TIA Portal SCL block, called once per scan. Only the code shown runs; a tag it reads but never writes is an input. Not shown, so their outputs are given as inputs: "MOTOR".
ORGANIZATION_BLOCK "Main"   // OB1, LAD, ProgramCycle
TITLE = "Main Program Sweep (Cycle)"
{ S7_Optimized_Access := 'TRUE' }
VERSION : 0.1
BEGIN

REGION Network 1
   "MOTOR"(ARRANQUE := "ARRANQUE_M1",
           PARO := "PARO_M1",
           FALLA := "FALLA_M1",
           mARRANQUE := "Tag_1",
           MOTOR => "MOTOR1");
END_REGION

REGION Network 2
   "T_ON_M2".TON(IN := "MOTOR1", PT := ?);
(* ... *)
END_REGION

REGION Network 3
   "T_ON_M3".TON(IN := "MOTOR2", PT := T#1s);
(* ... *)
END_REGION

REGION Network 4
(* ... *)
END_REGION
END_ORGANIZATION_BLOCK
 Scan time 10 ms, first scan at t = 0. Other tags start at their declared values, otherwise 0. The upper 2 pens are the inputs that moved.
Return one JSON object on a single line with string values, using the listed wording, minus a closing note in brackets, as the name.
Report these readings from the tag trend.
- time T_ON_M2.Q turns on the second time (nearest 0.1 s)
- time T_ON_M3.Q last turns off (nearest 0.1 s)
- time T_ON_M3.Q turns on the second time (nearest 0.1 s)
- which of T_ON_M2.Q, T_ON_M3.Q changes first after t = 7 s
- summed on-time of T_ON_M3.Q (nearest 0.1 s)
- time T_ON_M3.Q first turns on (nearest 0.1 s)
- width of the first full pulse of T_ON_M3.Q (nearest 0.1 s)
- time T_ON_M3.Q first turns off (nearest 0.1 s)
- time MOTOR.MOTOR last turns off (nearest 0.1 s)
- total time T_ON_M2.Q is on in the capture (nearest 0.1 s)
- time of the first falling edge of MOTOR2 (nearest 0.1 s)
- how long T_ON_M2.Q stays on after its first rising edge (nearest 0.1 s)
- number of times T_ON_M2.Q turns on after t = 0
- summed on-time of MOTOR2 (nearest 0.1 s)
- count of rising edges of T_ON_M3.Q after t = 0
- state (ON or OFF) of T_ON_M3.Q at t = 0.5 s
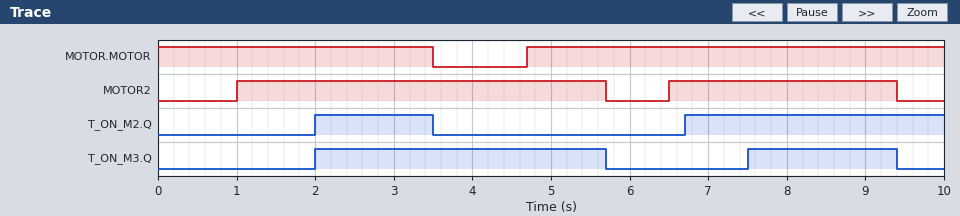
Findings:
{"time T_ON_M2.Q turns on the second time": "6.7 s", "time T_ON_M3.Q last turns off": "9.4 s", "time T_ON_M3.Q turns on the second time": "7.5 s", "which of T_ON_M2.Q, T_ON_M3.Q changes first after t = 7 s": "T_ON_M3.Q", "summed on-time of T_ON_M3.Q": "5.6 s", "time T_ON_M3.Q first turns on": "2.0 s", "width of the first full pulse of T_ON_M3.Q": "3.7 s", "time T_ON_M3.Q first turns off": "5.7 s", "time MOTOR.MOTOR last turns off": "3.5 s", "total time T_ON_M2.Q is on in the capture": "4.8 s", "time of the first falling edge of MOTOR2": "5.7 s", "how long T_ON_M2.Q stays on after its first rising edge": "1.5 s", "number of times T_ON_M2.Q turns on after t = 0": "2", "summed on-time of MOTOR2": "7.6 s", "count of rising edges of T_ON_M3.Q after t = 0": "2", "state (ON or OFF) of T_ON_M3.Q at t = 0.5 s": "OFF"}
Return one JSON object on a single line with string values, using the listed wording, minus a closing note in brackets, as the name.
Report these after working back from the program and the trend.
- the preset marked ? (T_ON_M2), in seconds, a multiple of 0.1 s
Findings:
{"the preset marked ? (T_ON_M2), in seconds, a multiple of 0.1 s": "2.0 s"}
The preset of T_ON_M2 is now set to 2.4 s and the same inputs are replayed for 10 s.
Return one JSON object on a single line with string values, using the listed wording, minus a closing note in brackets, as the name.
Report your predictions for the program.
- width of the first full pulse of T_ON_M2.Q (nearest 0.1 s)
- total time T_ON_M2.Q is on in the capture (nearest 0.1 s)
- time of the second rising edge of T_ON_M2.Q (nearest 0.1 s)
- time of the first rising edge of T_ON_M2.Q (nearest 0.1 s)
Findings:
{"width of the first full pulse of T_ON_M2.Q": "1.1 s", "total time T_ON_M2.Q is on in the capture": "4.0 s", "time of the second rising edge of T_ON_M2.Q": "7.1 s", "time of the first rising edge of T_ON_M2.Q": "2.4 s"}
